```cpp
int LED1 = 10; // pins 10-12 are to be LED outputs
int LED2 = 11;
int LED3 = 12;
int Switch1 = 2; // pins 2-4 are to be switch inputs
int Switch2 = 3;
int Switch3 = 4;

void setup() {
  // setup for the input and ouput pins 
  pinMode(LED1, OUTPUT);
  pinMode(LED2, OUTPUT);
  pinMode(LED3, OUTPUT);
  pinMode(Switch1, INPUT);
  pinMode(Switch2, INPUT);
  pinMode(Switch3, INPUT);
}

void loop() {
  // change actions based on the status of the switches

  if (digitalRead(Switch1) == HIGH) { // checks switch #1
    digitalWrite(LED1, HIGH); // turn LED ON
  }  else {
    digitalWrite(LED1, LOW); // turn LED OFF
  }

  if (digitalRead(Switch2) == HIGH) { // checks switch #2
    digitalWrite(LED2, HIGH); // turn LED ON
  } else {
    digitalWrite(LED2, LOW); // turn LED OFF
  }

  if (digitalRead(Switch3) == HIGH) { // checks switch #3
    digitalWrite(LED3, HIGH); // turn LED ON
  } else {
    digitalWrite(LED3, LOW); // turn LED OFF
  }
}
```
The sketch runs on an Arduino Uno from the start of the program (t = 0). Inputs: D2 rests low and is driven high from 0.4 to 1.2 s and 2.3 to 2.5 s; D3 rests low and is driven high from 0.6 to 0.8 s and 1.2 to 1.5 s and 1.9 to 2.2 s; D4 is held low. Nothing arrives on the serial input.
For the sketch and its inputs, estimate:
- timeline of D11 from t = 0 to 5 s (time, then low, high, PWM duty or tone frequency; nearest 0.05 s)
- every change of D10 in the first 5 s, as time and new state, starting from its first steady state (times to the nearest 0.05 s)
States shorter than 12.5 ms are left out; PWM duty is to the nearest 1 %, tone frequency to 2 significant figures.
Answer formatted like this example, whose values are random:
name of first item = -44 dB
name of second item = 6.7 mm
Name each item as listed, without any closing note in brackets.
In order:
timeline of D11 from t = 0 to 5 s = 0 s low; 0.6 s high; 0.8 s low; 1.2 s high; 1.5 s low; 1.9 s high; 2.2 s low
every change of D10 in the first 5 s, as time and new state, starting from its first steady state = 0 s low; 0.4 s high; 1.2 s low; 2.3 s high; 2.5 s low
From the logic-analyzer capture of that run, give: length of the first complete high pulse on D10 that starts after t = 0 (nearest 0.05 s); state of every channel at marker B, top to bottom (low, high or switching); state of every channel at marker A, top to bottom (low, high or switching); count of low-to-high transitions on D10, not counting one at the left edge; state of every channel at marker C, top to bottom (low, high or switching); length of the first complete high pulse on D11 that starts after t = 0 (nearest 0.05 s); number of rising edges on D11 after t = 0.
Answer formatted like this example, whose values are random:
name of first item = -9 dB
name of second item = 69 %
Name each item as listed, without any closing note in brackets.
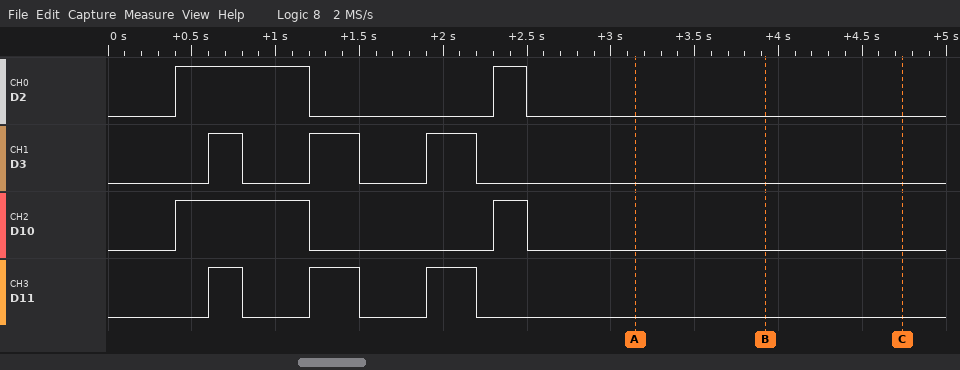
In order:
length of the first complete high pulse on D10 that starts after t = 0 = 0.80 s
state of every channel at marker B, top to bottom = D2 low, D3 low, D10 low, D11 low
state of every channel at marker A, top to bottom = D2 low, D3 low, D10 low, D11 low
count of low-to-high transitions on D10, not counting one at the left edge = 2
state of every channel at marker C, top to bottom = D2 low, D3 low, D10 low, D11 low
length of the first complete high pulse on D11 that starts after t = 0 = 0.20 s
number of rising edges on D11 after t = 0 = 3
